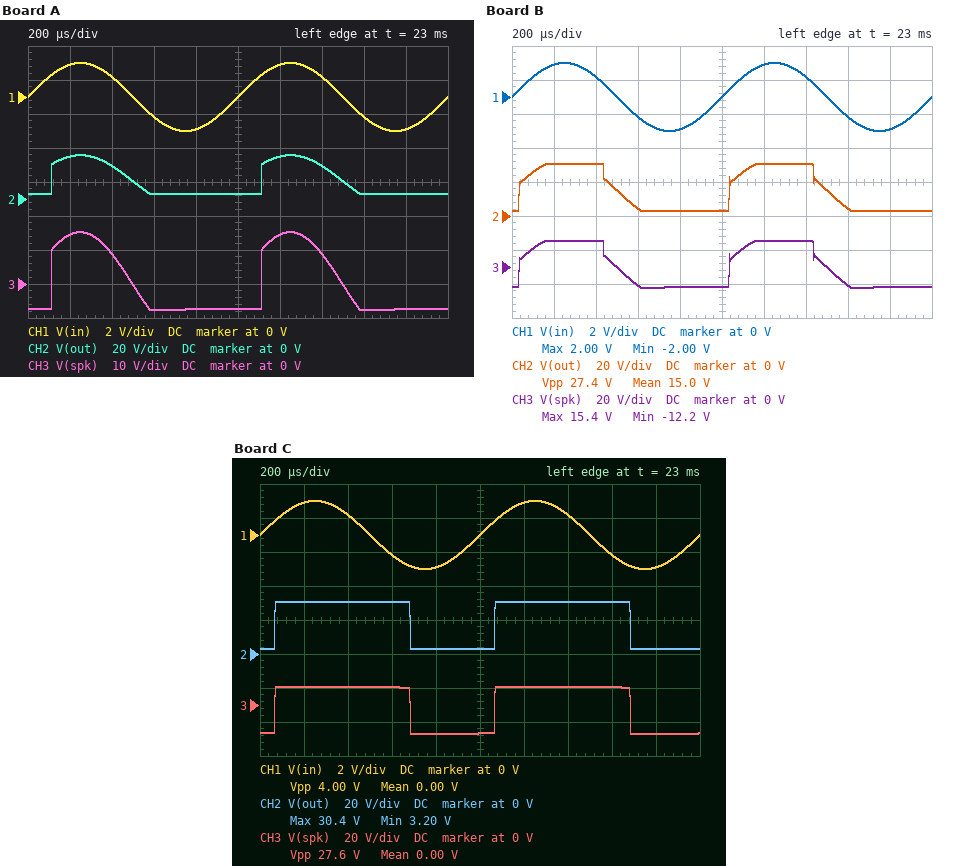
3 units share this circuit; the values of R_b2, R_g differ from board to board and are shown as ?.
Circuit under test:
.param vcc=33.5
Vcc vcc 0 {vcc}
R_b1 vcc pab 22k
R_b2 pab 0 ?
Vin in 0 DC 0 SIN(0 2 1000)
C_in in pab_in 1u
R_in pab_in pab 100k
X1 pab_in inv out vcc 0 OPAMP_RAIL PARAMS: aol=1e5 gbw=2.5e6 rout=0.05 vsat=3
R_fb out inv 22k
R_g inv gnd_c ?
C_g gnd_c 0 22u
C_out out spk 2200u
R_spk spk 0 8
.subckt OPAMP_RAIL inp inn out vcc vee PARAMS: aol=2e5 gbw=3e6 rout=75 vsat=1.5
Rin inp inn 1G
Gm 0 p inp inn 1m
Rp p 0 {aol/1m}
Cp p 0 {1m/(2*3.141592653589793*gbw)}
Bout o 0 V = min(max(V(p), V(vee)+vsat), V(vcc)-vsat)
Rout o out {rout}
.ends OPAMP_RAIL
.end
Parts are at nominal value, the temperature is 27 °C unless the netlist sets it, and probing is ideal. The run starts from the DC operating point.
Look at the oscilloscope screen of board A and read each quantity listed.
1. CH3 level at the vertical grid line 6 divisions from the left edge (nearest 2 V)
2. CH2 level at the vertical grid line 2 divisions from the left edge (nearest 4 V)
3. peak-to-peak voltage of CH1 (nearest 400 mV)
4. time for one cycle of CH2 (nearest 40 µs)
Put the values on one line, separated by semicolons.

14 V; 20 V; 4.0 V; 1.00 ms
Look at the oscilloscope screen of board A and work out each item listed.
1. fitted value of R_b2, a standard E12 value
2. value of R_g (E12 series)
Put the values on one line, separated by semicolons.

10 kΩ; 3.3 kΩ
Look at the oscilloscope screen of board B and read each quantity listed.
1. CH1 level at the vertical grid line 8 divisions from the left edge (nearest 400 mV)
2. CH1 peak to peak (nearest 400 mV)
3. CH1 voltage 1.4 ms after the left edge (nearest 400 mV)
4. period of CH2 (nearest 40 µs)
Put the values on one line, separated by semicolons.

-1.2 V; 4.0 V; 1.2 V; 1.00 ms
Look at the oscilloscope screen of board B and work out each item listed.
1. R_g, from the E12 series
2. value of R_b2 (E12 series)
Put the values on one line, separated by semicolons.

2.7 kΩ; 18 kΩ
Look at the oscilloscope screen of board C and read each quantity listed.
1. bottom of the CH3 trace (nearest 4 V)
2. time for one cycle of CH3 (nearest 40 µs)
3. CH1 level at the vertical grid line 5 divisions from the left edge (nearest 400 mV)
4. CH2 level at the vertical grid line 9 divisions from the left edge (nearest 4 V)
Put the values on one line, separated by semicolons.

-16 V; 1.00 ms; 0 V; 4 V
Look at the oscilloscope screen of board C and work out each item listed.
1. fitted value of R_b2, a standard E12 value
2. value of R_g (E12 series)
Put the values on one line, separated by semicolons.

33 kΩ; 1.5 kΩ
